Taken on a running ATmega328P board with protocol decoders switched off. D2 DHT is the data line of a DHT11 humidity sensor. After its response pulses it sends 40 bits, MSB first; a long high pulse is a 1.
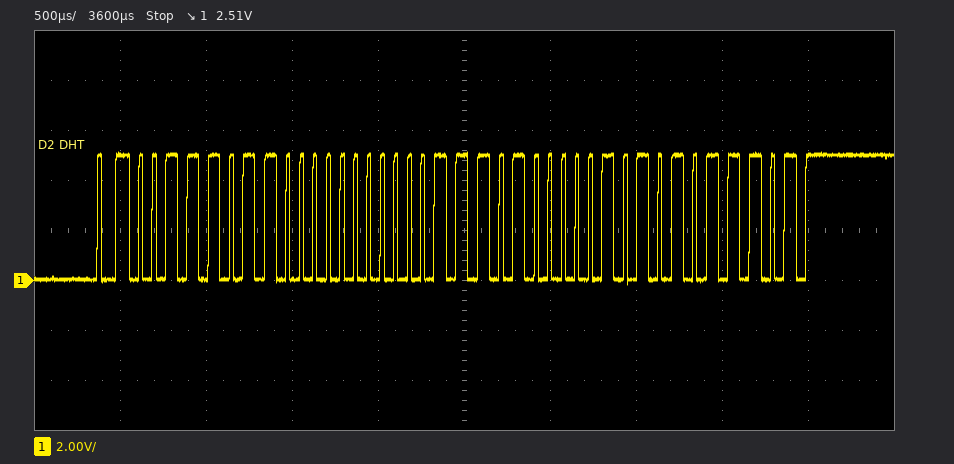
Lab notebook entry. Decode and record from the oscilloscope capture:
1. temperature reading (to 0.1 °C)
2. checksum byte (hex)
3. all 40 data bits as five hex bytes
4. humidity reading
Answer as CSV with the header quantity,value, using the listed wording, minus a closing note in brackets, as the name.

quantity,value
temperature reading,29.5 °C
checksum byte,0x5D
all 40 data bits as five hex bytes,3B 00 1D 05 5D
humidity reading,59 %
